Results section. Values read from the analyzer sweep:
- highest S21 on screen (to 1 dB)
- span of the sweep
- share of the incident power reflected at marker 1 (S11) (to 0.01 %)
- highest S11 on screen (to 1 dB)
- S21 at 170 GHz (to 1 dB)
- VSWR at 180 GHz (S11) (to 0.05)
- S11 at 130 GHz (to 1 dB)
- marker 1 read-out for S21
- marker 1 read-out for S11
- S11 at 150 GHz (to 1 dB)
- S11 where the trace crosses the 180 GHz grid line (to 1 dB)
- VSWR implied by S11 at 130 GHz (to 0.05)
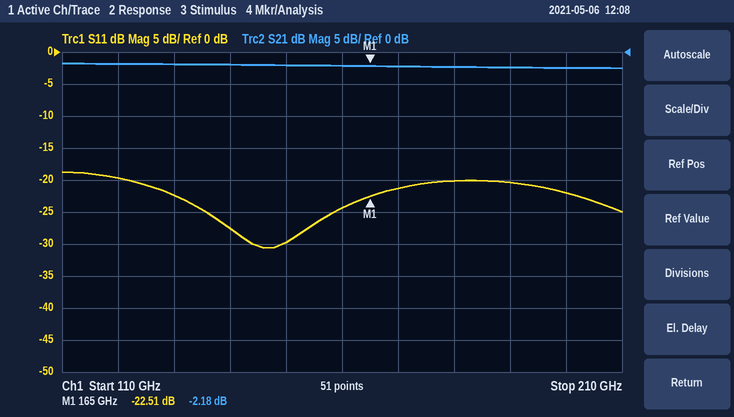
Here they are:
-2 dB
100 GHz
0.56 %
-19 dB
-2 dB
1.20
-22 dB
-2.18 dB
-22.51 dB
-30 dB
-20 dB
1.15
